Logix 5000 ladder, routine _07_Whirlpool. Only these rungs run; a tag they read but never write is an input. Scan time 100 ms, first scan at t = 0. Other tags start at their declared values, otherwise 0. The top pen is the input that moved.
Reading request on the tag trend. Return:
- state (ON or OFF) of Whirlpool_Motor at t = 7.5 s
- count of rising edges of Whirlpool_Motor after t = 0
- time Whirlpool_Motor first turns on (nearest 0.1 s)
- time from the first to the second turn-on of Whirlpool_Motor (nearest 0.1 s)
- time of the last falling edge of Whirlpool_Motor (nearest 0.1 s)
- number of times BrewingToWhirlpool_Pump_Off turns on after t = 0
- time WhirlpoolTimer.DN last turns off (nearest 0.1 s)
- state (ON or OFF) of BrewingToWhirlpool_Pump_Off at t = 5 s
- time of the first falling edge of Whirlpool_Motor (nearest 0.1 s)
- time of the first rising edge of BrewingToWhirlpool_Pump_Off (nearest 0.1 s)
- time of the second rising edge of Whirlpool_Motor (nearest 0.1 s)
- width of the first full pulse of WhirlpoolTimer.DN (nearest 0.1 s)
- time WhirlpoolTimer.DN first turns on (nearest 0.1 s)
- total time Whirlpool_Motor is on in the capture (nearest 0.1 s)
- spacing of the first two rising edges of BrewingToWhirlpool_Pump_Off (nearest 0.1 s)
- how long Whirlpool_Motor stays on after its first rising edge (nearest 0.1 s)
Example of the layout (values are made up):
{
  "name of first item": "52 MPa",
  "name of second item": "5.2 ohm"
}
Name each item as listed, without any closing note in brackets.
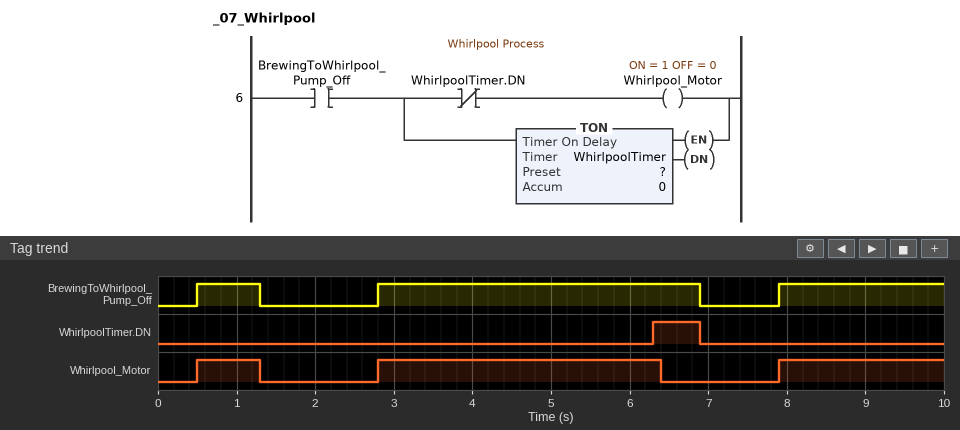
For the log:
{
  "state (ON or OFF) of Whirlpool_Motor at t = 7.5 s": "OFF",
  "count of rising edges of Whirlpool_Motor after t = 0": "3",
  "time Whirlpool_Motor first turns on": "0.5 s",
  "time from the first to the second turn-on of Whirlpool_Motor": "2.3 s",
  "time of the last falling edge of Whirlpool_Motor": "6.4 s",
  "number of times BrewingToWhirlpool_Pump_Off turns on after t = 0": "3",
  "time WhirlpoolTimer.DN last turns off": "6.9 s",
  "state (ON or OFF) of BrewingToWhirlpool_Pump_Off at t = 5 s": "ON",
  "time of the first falling edge of Whirlpool_Motor": "1.3 s",
  "time of the first rising edge of BrewingToWhirlpool_Pump_Off": "0.5 s",
  "time of the second rising edge of Whirlpool_Motor": "2.8 s",
  "width of the first full pulse of WhirlpoolTimer.DN": "0.6 s",
  "time WhirlpoolTimer.DN first turns on": "6.3 s",
  "total time Whirlpool_Motor is on in the capture": "6.5 s",
  "spacing of the first two rising edges of BrewingToWhirlpool_Pump_Off": "2.3 s",
  "how long Whirlpool_Motor stays on after its first rising edge": "0.8 s"
}
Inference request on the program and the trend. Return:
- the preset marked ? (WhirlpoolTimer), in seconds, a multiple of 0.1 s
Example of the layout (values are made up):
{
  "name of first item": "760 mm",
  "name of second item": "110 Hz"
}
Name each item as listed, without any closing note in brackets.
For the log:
{
  "the preset marked ? (WhirlpoolTimer), in seconds, a multiple of 0.1 s": "3.5 s"
}
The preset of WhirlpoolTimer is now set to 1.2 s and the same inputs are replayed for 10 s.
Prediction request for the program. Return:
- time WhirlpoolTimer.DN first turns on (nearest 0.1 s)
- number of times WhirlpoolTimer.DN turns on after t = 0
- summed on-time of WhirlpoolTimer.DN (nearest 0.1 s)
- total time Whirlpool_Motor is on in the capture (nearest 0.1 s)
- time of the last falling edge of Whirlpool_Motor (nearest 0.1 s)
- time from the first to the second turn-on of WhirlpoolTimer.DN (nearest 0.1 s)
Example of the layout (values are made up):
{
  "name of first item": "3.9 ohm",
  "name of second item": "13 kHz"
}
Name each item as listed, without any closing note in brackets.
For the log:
{
  "time WhirlpoolTimer.DN first turns on": "4.0 s",
  "number of times WhirlpoolTimer.DN turns on after t = 0": "2",
  "summed on-time of WhirlpoolTimer.DN": "3.8 s",
  "total time Whirlpool_Motor is on in the capture": "3.4 s",
  "time of the last falling edge of Whirlpool_Motor": "9.2 s",
  "time from the first to the second turn-on of WhirlpoolTimer.DN": "5.1 s"
}
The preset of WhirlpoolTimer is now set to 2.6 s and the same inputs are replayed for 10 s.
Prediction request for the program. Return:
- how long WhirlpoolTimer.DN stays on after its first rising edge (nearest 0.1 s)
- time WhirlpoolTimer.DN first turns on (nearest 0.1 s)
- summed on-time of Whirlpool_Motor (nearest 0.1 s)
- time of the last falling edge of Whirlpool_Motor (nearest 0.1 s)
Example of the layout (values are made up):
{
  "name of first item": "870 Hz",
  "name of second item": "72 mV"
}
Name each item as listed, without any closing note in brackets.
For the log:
{
  "how long WhirlpoolTimer.DN stays on after its first rising edge": "1.5 s",
  "time WhirlpoolTimer.DN first turns on": "5.4 s",
  "summed on-time of Whirlpool_Motor": "5.6 s",
  "time of the last falling edge of Whirlpool_Motor": "5.5 s"
}
